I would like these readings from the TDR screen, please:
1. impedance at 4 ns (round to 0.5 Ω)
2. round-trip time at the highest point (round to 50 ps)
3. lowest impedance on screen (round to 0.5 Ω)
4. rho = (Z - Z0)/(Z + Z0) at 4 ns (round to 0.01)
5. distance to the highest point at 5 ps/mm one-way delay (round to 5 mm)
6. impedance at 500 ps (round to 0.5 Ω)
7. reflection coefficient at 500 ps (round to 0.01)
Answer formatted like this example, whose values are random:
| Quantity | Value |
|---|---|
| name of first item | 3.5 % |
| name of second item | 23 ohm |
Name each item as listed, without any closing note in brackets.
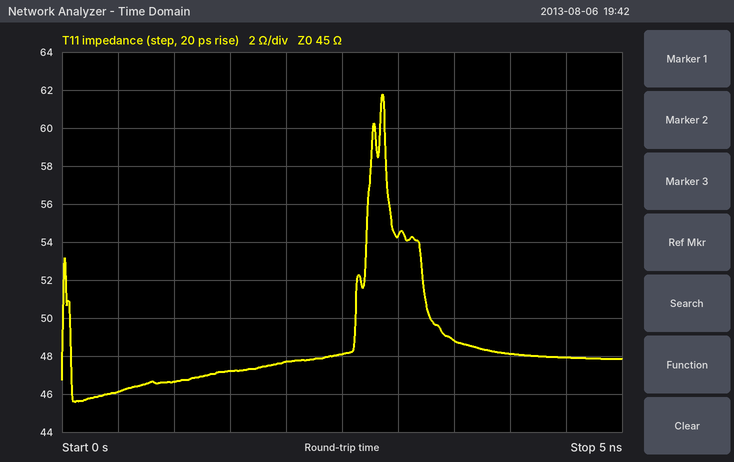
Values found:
| Quantity | Value |
|---|---|
| impedance at 4 ns | 48.0 Ω |
| round-trip time at the highest point | 2.85 ns |
| lowest impedance on screen | 45.5 Ω |
| rho = (Z - Z0)/(Z + Z0) at 4 ns | +0.03 |
| distance to the highest point at 5 ps/mm one-way delay | 285 mm |
| impedance at 500 ps | 46.0 Ω |
| reflection coefficient at 500 ps | +0.01 |
